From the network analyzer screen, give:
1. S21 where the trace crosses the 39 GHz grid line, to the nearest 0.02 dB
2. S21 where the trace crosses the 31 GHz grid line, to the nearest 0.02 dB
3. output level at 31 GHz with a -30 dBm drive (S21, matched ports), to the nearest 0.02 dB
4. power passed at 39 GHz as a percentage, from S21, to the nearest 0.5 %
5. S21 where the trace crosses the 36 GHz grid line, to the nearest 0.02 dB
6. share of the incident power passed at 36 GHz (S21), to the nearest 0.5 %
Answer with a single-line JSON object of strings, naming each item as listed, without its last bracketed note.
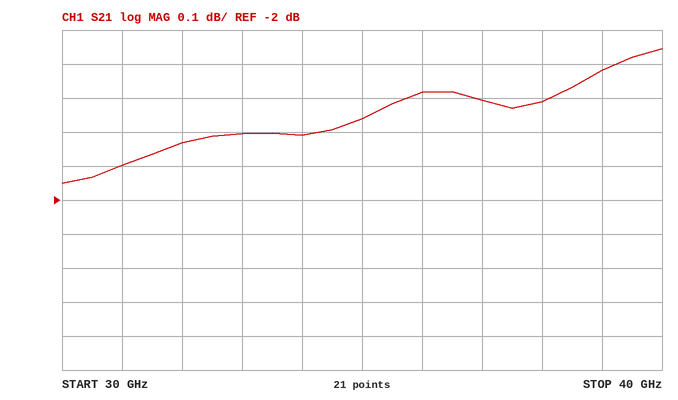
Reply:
{"S21 where the trace crosses the 39 GHz grid line, to the nearest 0.02 dB": "-1.62 dB", "S21 where the trace crosses the 31 GHz grid line, to the nearest 0.02 dB": "-1.90 dB", "output level at 31 GHz with a -30 dBm drive (S21, matched ports), to the nearest 0.02 dB": "-31.90 dBm", "power passed at 39 GHz as a percentage, from S21, to the nearest 0.5 %": "69.0 %", "S21 where the trace crosses the 36 GHz grid line, to the nearest 0.02 dB": "-1.68 dB", "share of the incident power passed at 36 GHz (S21), to the nearest 0.5 %": "68.0 %"}
